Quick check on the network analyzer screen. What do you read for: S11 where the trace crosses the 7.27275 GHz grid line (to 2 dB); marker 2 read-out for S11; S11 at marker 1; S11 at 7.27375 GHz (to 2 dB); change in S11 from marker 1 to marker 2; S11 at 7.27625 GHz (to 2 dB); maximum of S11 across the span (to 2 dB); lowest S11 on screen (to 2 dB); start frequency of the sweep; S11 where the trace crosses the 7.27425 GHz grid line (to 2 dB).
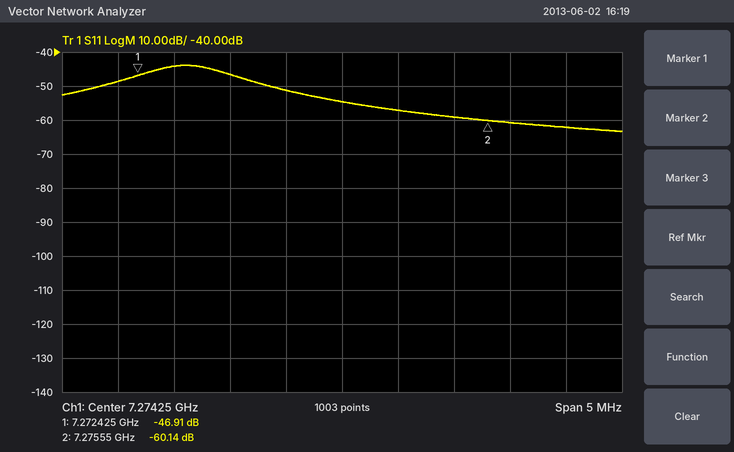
-44 dB
-60.14 dB
-46.91 dB
-52 dB
-13.23 dB
-62 dB
-44 dB
-64 dB
7.27175 GHz
-54 dB
